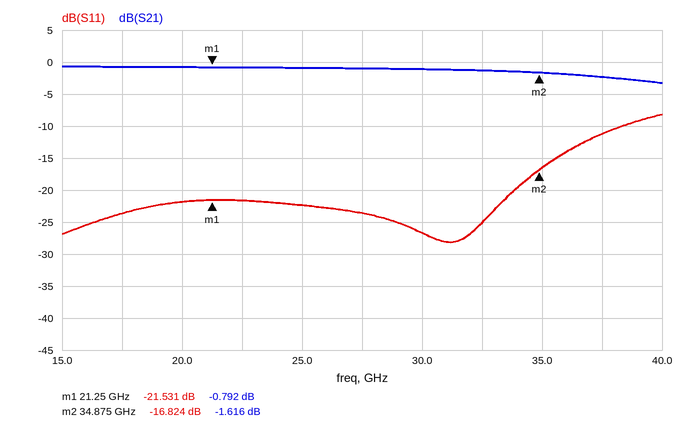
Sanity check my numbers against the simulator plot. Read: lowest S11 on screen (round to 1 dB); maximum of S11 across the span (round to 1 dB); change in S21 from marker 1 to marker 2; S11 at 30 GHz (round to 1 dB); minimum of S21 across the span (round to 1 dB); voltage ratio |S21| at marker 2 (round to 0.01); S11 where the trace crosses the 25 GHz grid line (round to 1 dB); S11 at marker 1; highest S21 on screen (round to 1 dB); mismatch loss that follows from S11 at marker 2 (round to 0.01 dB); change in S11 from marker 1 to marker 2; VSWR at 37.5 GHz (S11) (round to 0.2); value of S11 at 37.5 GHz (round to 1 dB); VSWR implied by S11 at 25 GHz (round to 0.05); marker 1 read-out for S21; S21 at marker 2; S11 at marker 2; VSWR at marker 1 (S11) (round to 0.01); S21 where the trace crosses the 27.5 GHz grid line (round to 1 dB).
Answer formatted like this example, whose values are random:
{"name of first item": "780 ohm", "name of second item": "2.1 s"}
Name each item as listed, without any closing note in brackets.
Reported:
{"lowest S11 on screen": "-28 dB", "maximum of S11 across the span": "-8 dB", "change in S21 from marker 1 to marker 2": "-0.824 dB", "S11 at 30 GHz": "-27 dB", "minimum of S21 across the span": "-3 dB", "voltage ratio |S21| at marker 2": "0.83", "S11 where the trace crosses the 25 GHz grid line": "-22 dB", "S11 at marker 1": "-21.531 dB", "highest S21 on screen": "-1 dB", "mismatch loss that follows from S11 at marker 2": "0.09 dB", "change in S11 from marker 1 to marker 2": "4.707 dB", "VSWR at 37.5 GHz (S11)": "1.8", "value of S11 at 37.5 GHz": "-11 dB", "VSWR implied by S11 at 25 GHz": "1.15", "marker 1 read-out for S21": "-0.792 dB", "S21 at marker 2": "-1.616 dB", "S11 at marker 2": "-16.824 dB", "VSWR at marker 1 (S11)": "1.18", "S21 where the trace crosses the 27.5 GHz grid line": "-1 dB"}
